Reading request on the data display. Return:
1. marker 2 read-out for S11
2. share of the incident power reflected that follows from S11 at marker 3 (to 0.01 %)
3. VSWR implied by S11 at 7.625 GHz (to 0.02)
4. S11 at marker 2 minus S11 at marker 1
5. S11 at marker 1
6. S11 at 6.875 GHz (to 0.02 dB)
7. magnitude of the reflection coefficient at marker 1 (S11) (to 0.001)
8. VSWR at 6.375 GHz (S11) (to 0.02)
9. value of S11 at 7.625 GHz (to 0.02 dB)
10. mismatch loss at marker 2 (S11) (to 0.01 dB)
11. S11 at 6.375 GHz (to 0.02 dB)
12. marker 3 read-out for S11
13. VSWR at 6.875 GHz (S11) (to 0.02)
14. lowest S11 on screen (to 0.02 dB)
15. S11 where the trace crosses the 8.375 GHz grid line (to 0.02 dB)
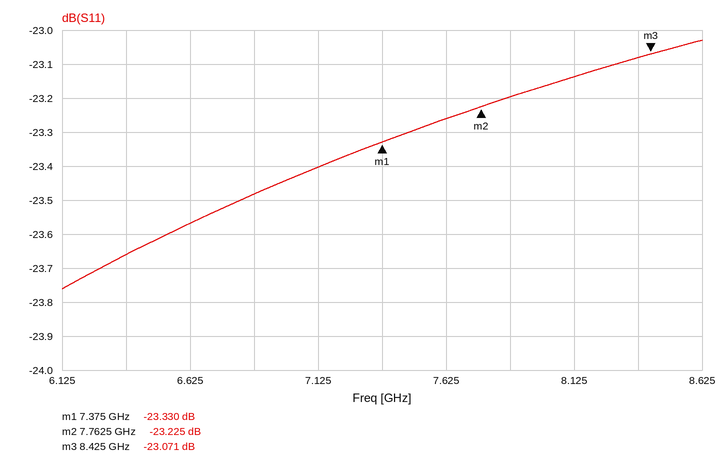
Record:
-23.225 dB
0.49 %
1.14
0.105 dB
-23.330 dB
-23.48 dB
0.068
1.14
-23.26 dB
0.02 dB
-23.66 dB
-23.071 dB
1.14
-23.76 dB
-23.08 dB
